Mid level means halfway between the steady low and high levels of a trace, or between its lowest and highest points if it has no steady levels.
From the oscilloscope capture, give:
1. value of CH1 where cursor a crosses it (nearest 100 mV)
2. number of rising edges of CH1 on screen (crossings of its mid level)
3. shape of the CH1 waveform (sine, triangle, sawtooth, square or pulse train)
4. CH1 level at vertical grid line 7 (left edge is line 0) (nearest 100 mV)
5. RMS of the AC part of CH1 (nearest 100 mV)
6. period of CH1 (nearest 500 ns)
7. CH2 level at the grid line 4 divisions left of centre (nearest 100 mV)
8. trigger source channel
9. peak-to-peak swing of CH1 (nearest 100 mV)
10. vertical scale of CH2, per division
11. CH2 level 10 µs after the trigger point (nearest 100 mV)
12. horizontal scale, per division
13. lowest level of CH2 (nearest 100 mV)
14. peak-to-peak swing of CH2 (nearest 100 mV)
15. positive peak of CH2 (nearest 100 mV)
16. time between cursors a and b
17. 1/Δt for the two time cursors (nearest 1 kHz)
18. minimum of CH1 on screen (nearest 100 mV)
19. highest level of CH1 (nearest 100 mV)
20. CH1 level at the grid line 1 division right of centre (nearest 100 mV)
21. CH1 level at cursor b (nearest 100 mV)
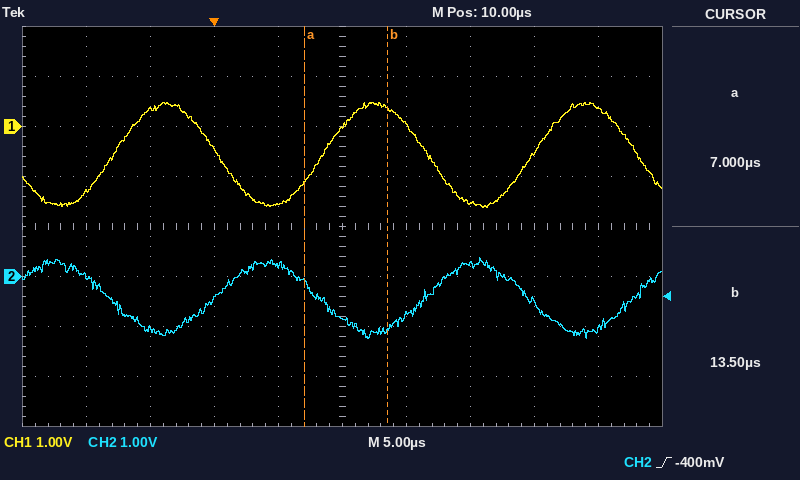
-1.1 V
3
sine
-1.5 V
700 mV
16.5 µs
0.0 V
CH2
2.1 V
1 V
-800 mV
5 µs
-1.2 V
1.6 V
400 mV
6.5 µs
154 kHz
-1.6 V
500 mV
0.0 V
400 mV
